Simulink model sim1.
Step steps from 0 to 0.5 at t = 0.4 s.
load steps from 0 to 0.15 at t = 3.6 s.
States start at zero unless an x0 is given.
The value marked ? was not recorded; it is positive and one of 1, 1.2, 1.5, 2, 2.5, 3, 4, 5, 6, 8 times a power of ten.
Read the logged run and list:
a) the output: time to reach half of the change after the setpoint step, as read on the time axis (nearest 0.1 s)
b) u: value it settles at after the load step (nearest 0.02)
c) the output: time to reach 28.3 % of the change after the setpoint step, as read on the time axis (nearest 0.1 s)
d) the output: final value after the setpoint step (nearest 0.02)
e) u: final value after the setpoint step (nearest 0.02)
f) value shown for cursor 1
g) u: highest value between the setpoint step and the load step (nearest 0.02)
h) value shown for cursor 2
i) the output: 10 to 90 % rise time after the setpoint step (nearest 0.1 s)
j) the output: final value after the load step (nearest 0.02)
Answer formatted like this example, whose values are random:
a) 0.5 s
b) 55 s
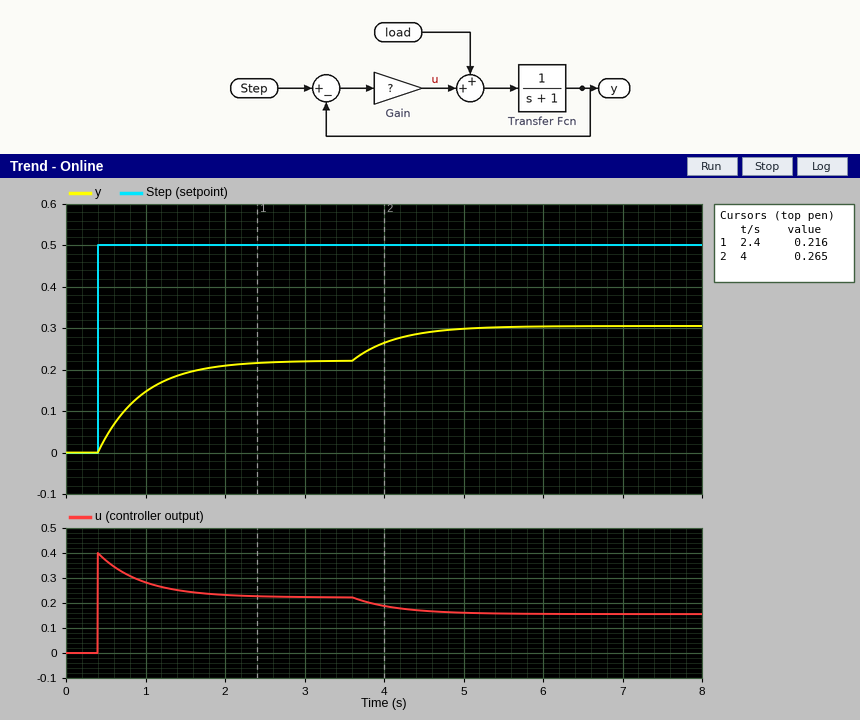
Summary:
a) 0.8 s
b) 0.16
c) 0.6 s
d) 0.22
e) 0.22
f) 0.216
g) 0.40
h) 0.265
i) 1.2 s
j) 0.30
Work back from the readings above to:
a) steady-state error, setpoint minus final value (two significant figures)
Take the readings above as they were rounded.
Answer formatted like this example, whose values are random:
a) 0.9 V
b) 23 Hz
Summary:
a) 0.28
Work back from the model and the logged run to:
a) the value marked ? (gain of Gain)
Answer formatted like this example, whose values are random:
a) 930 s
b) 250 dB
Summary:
a) 0.8
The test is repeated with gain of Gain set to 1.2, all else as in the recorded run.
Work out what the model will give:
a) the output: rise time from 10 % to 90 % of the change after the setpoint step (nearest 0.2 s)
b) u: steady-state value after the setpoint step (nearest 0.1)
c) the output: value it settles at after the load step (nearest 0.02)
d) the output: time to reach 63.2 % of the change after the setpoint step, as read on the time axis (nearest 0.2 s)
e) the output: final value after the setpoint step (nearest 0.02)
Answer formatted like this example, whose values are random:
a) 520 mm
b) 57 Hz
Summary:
a) 1.0 s
b) 0.3
c) 0.34
d) 0.8 s
e) 0.28
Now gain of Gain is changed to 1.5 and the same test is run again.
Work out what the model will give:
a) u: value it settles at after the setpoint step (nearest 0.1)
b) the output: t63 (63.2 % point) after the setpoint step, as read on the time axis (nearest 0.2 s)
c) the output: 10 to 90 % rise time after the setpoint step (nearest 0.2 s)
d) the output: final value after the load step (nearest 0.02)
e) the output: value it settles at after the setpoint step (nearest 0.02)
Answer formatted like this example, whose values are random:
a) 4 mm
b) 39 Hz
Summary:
a) 0.3
b) 0.8 s
c) 0.8 s
d) 0.36
e) 0.30
